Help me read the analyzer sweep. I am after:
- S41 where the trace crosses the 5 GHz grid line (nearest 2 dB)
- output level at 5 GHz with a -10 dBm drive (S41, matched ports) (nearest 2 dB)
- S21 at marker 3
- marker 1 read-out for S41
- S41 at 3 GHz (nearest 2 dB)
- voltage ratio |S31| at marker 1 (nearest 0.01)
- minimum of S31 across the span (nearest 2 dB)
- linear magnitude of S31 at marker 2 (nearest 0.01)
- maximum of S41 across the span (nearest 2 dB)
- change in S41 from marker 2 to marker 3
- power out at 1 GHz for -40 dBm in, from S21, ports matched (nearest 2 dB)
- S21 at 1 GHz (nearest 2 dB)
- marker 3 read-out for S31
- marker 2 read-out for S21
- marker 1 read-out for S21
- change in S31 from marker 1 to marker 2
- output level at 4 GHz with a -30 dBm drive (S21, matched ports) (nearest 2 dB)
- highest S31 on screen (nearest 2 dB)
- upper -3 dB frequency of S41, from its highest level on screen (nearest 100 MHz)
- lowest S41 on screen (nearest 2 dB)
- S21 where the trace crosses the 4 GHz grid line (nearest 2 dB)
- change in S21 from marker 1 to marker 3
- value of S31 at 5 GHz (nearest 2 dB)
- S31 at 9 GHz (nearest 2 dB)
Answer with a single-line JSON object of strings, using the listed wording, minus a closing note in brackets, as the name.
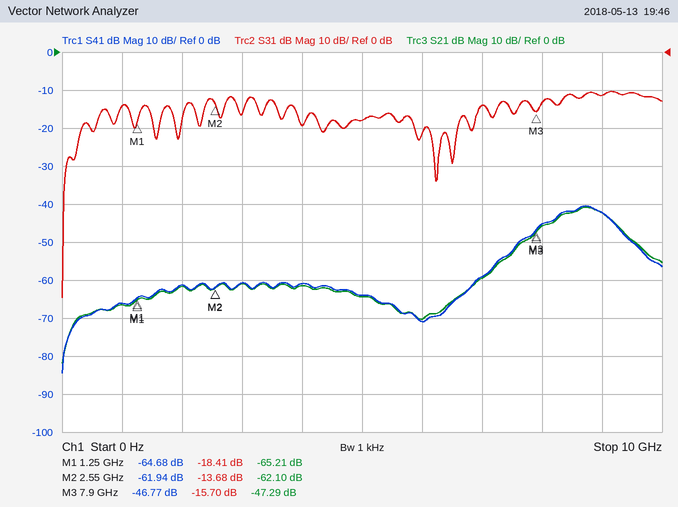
{"S41 where the trace crosses the 5 GHz grid line": "-64 dB", "output level at 5 GHz with a -10 dBm drive (S41, matched ports)": "-74 dBm", "S21 at marker 3": "-47.29 dB", "marker 1 read-out for S41": "-64.68 dB", "S41 at 3 GHz": "-60 dB", "voltage ratio |S31| at marker 1": "0.12", "minimum of S31 across the span": "-64 dB", "linear magnitude of S31 at marker 2": "0.21", "maximum of S41 across the span": "-40 dB", "change in S41 from marker 2 to marker 3": "15.17 dB", "power out at 1 GHz for -40 dBm in, from S21, ports matched": "-106 dBm", "S21 at 1 GHz": "-66 dB", "marker 3 read-out for S31": "-15.70 dB", "marker 2 read-out for S21": "-62.10 dB", "marker 1 read-out for S21": "-65.21 dB", "change in S31 from marker 1 to marker 2": "4.73 dB", "output level at 4 GHz with a -30 dBm drive (S21, matched ports)": "-92 dBm", "highest S31 on screen": "-10 dB", "upper -3 dB frequency of S41, from its highest level on screen": "9.1 GHz", "lowest S41 on screen": "-84 dB", "S21 where the trace crosses the 4 GHz grid line": "-62 dB", "change in S21 from marker 1 to marker 3": "17.92 dB", "value of S31 at 5 GHz": "-18 dB", "S31 at 9 GHz": "-12 dB"}
